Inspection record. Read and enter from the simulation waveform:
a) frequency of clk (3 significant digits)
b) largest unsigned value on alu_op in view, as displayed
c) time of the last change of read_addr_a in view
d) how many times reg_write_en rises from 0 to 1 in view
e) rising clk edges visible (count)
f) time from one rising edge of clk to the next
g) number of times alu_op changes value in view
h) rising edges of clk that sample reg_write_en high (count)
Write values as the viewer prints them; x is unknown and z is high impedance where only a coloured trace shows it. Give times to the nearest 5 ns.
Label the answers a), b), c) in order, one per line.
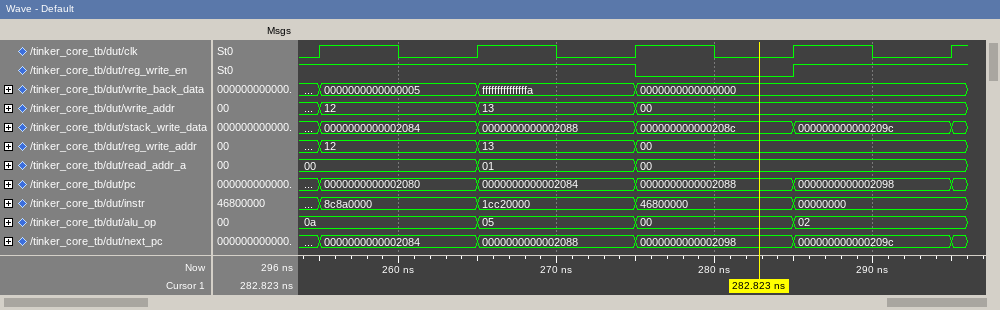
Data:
a) 100 MHz
b) 0a
c) 275 ns
d) 1
e) 5
f) 10 ns
g) 3
h) 4
